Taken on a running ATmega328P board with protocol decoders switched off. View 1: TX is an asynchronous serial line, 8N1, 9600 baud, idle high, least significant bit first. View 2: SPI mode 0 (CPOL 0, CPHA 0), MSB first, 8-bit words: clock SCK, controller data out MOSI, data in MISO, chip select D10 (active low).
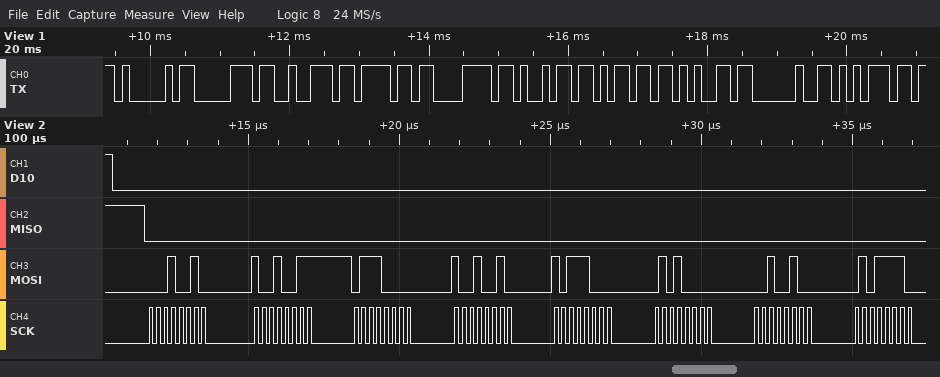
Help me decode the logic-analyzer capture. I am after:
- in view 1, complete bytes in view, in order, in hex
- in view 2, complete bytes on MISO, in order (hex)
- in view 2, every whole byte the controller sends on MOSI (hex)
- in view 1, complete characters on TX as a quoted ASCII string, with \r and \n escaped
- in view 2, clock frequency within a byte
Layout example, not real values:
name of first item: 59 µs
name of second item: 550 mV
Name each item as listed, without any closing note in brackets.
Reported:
in view 1, complete bytes in view, in order, in hex: 41 70 72 6F 78 69 6D 65 20 75
in view 2, complete bytes on MISO, in order: 0x00 0x00 0x00 0x00 0x00 0x00 0x00 0x00
in view 2, every whole byte the controller sends on MOSI: 0x12 0x93 0x70 0x92 0xB8 0x50 0x24 0x5E
in view 1, complete characters on TX as a quoted ASCII string, with \r and \n escaped: "Aproxime u"
in view 2, clock frequency within a byte: 4 MHz
